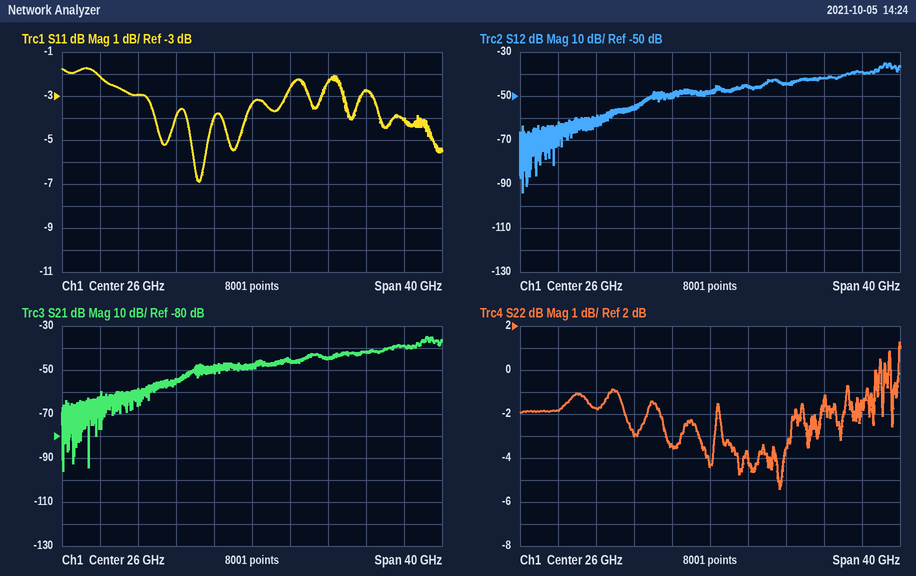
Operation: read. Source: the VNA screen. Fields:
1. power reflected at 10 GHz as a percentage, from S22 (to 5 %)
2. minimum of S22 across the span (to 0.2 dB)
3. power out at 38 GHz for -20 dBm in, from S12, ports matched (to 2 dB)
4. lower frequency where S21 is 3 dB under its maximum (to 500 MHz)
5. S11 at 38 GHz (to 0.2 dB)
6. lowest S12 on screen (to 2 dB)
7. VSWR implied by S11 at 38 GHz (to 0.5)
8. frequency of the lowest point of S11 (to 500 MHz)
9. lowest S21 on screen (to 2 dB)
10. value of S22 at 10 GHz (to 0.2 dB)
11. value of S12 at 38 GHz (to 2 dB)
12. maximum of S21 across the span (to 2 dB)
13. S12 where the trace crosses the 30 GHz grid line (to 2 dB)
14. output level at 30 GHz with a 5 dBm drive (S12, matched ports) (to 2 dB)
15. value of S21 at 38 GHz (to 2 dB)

65 %
-5.4 dB
-62 dBm
44.0 GHz
-2.8 dB
-94 dB
6.5
20.5 GHz
-96 dB
-1.8 dB
-42 dB
-34 dB
-46 dB
-40 dBm
-42 dB
